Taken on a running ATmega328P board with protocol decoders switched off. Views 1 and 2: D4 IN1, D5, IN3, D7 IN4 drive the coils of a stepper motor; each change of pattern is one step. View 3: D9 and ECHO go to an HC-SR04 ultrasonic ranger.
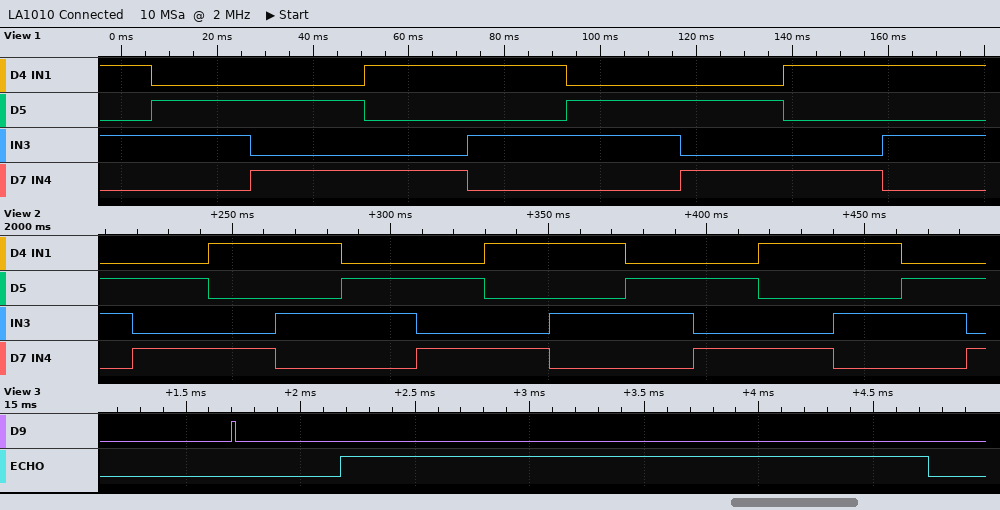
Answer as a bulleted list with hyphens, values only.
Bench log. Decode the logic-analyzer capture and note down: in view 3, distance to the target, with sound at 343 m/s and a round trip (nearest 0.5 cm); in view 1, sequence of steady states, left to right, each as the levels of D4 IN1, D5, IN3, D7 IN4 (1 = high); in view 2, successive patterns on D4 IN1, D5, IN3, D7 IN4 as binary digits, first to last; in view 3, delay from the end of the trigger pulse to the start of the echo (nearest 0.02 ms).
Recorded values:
- 44 cm
- 1010 0110 0101 1001 1010 0110 0101 1001 1010
- 0110 0101 1001 1010 0110 0101 1001 1010 0110 0101 1001 1010 0110 0101
- 0.46 ms
